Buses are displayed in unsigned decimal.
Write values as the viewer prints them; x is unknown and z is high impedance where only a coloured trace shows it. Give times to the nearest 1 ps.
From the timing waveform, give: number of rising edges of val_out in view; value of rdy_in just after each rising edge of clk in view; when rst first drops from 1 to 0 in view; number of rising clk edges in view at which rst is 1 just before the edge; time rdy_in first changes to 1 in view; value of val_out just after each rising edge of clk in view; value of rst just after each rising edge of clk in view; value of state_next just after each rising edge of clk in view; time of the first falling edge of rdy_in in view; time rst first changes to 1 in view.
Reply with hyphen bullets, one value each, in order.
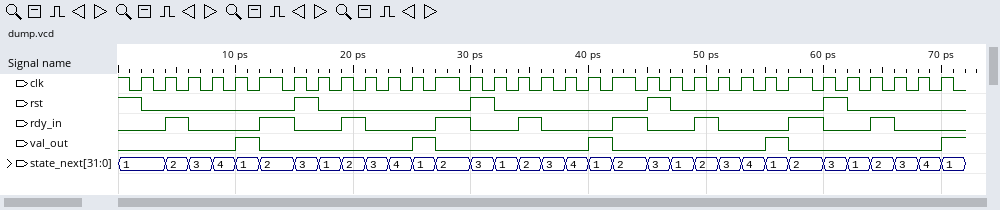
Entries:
- 5
- 0 1 0 0 0 1 0 0 1 0 0 0 1 0 0 1 0 0 0 1 0 0 1 0 0 0 1 0 0 1 0 0 0
- 2 ps
- 5
- 4 ps
- 0 0 0 0 1 0 0 0 0 0 0 1 0 0 0 0 0 0 1 0 0 0 0 0 0 1 0 0 0 0 0 0 1
- 0 0 0 0 0 0 1 0 0 0 0 0 0 1 0 0 0 0 0 0 1 0 0 0 0 0 0 1 0 0 0 0 0
- 1, 2, 3, 4, 1, 2, 3, 1, 2, 3, 4, 1, 2, 3, 1, 2, 3, 4, 1, 2, 3, 1, 2, 3, 4, 1, 2, 3, 1, 2, 3, 4, 1
- 6 ps
- 15 ps
